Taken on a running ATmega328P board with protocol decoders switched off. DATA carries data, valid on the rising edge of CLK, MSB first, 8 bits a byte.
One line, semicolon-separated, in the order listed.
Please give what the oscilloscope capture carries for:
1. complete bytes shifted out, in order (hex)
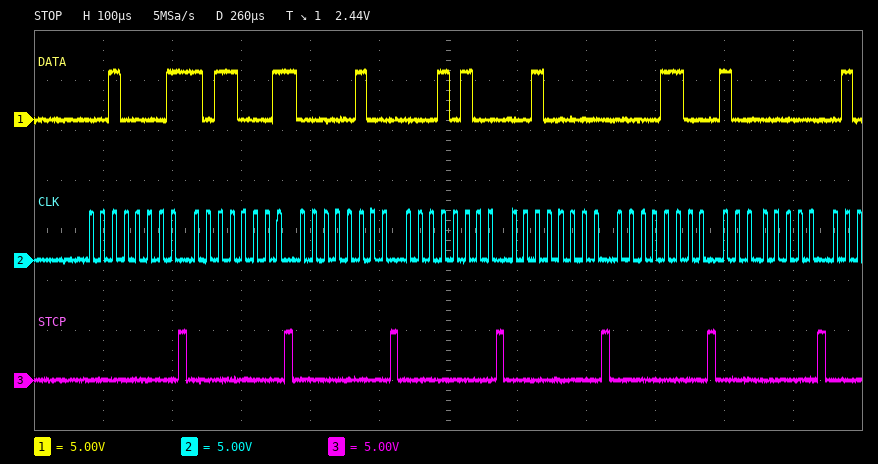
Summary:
0x21 0xB1 0x04 0x14 0x20 0x0C 0x80
